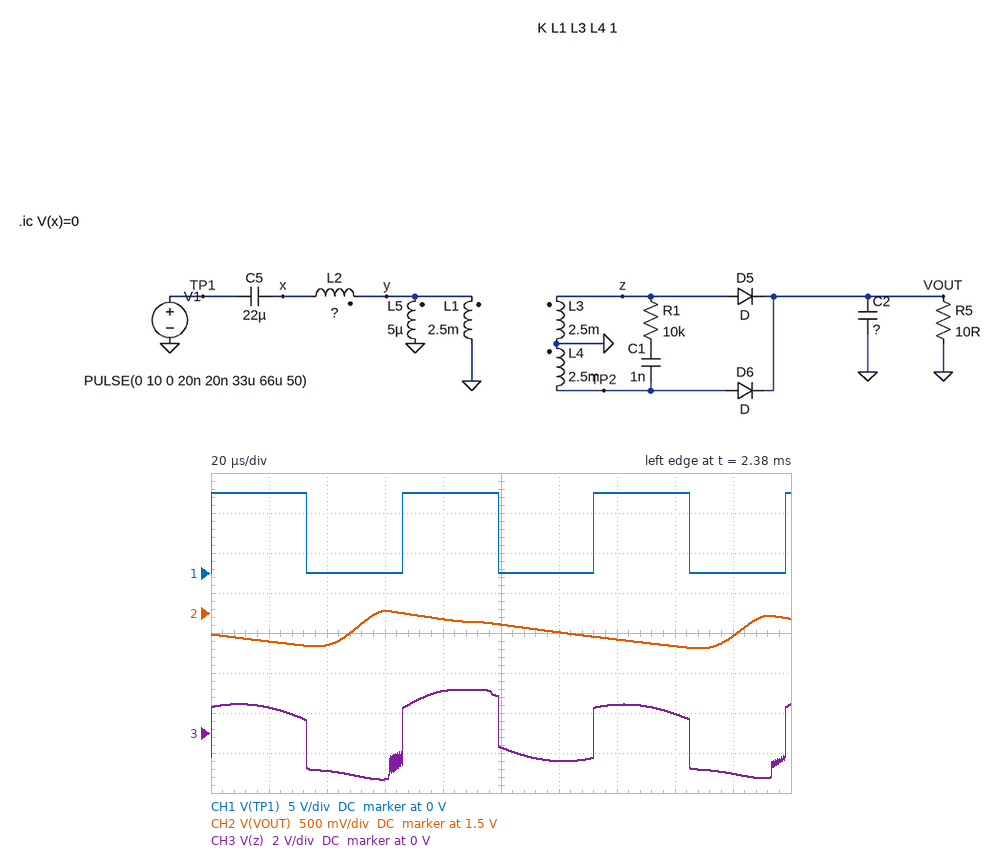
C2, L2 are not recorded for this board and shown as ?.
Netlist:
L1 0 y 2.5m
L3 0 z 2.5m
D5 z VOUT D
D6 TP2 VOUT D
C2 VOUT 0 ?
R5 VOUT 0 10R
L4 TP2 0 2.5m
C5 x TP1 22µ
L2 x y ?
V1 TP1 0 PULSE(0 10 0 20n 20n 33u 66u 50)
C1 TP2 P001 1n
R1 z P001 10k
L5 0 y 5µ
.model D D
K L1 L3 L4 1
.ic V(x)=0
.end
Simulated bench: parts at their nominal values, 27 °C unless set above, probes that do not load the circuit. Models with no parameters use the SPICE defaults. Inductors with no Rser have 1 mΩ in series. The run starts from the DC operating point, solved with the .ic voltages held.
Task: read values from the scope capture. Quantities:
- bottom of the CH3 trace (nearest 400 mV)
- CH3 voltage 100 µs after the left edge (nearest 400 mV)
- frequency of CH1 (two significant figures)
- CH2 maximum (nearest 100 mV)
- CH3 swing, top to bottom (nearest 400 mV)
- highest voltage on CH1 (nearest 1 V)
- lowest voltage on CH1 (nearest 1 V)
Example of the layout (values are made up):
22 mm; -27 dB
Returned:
-2.4 V; -800 mV; 15 kHz; 1.5 V; 4.4 V; 10 V; 0 V
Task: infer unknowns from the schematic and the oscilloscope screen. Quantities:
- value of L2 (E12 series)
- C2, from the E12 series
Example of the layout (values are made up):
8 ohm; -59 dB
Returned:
15 µH; 27 µF
